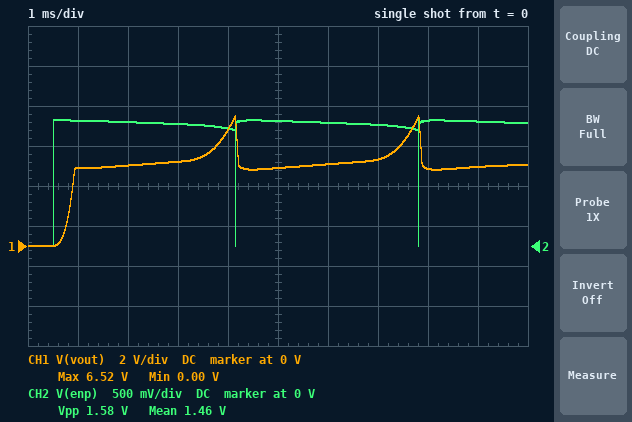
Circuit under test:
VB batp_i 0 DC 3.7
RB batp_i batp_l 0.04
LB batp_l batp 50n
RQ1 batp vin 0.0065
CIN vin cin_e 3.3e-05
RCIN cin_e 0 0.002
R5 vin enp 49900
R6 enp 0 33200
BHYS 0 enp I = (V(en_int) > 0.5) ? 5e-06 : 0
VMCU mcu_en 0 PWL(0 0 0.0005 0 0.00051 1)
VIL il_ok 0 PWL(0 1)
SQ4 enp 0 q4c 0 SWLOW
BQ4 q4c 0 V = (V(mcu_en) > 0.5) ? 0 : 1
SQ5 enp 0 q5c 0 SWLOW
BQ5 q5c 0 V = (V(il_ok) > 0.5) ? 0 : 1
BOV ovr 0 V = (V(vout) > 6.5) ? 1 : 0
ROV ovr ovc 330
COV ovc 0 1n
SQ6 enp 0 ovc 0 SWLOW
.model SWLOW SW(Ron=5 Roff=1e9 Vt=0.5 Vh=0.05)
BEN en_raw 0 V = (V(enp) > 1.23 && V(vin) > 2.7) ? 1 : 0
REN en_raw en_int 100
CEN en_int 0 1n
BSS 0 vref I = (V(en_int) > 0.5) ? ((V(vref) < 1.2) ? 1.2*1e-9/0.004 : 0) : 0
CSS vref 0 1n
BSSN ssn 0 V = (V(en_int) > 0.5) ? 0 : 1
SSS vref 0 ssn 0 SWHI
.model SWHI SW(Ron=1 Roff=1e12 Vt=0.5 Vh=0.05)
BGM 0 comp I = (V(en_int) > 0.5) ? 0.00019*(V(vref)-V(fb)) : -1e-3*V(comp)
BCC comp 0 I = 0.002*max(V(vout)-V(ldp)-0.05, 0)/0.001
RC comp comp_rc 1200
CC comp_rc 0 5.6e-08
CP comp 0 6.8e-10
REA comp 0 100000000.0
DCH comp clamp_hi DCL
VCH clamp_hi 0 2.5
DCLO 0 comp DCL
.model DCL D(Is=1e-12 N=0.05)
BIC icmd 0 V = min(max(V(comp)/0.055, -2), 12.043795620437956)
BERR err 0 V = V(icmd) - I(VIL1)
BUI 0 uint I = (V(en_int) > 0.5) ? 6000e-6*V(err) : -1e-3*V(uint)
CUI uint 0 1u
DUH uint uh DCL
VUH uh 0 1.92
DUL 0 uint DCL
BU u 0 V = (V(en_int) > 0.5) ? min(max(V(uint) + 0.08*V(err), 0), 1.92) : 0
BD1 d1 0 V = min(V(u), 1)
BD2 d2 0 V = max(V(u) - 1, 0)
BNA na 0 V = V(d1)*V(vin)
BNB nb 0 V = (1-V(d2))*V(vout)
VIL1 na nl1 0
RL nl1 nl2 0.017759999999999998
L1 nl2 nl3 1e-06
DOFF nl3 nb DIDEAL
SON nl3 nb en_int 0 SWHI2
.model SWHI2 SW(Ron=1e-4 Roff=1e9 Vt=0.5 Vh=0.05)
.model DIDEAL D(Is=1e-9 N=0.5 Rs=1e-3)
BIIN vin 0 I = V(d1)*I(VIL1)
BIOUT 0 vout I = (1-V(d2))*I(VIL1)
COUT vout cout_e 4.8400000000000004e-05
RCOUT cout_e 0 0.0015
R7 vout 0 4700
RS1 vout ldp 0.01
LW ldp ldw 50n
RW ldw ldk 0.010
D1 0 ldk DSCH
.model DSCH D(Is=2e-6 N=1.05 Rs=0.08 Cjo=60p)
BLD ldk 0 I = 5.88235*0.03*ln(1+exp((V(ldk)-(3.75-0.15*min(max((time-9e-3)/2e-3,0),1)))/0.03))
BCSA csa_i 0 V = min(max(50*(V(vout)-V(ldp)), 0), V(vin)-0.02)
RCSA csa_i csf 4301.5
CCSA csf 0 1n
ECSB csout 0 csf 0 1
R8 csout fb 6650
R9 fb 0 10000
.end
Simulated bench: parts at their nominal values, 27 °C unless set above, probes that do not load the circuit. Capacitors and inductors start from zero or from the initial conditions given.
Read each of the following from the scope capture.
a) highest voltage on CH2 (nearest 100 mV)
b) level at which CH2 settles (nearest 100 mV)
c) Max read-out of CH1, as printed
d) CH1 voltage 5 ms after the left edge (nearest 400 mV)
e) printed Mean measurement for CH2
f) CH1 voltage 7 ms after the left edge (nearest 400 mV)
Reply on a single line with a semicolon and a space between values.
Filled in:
1.6 V; 1.5 V; 6.52 V; 4.0 V; 1.46 V; 4.4 V
